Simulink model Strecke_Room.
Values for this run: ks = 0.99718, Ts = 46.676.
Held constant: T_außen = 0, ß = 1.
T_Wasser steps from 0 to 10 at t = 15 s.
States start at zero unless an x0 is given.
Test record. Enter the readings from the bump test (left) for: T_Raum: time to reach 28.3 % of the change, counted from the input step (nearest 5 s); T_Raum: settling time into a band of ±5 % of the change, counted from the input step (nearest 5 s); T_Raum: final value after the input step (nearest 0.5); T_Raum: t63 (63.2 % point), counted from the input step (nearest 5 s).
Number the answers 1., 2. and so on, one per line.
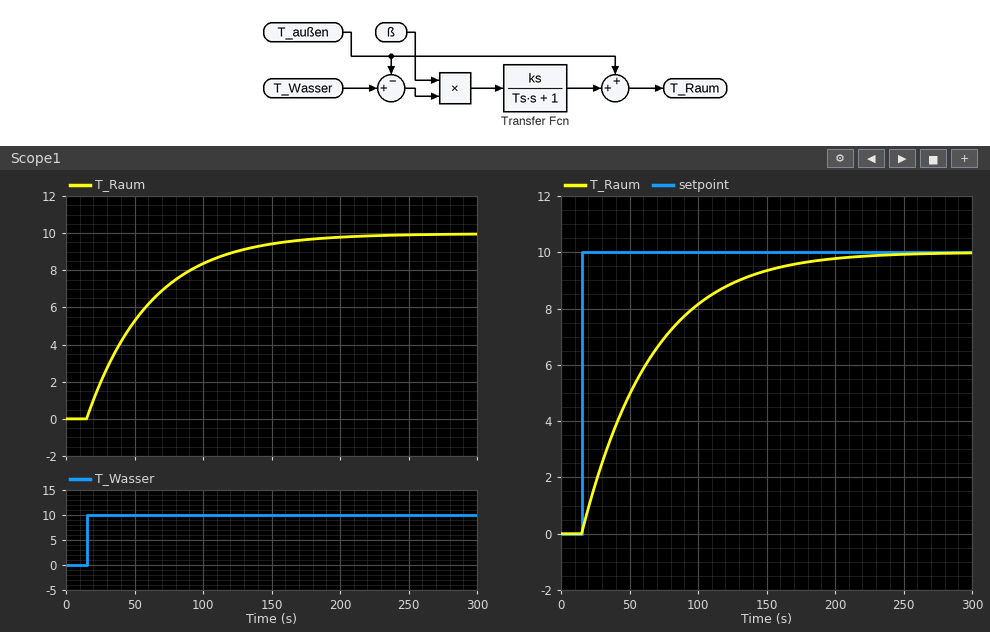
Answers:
1. 15 s
2. 140 s
3. 10.0
4. 45 s
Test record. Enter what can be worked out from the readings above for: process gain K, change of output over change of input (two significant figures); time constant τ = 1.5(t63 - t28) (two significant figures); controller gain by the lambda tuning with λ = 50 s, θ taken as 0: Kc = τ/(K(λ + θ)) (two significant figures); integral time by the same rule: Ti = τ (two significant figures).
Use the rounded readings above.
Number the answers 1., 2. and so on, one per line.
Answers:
1. 1.0
2. 45 s
3. 0.90
4. 45 s
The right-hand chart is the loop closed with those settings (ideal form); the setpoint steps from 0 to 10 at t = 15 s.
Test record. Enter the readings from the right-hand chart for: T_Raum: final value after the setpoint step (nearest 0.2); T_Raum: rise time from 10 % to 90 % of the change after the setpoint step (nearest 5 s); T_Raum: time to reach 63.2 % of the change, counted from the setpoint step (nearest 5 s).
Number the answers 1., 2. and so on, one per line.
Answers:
1. 10.0
2. 110 s
3. 50 s
